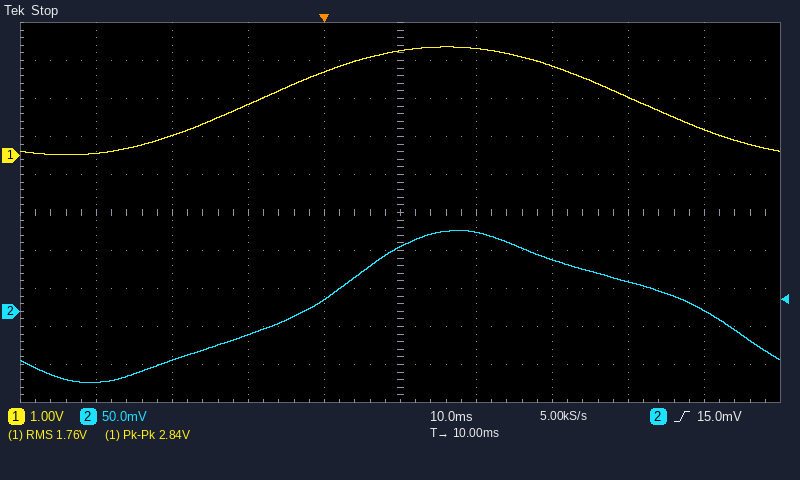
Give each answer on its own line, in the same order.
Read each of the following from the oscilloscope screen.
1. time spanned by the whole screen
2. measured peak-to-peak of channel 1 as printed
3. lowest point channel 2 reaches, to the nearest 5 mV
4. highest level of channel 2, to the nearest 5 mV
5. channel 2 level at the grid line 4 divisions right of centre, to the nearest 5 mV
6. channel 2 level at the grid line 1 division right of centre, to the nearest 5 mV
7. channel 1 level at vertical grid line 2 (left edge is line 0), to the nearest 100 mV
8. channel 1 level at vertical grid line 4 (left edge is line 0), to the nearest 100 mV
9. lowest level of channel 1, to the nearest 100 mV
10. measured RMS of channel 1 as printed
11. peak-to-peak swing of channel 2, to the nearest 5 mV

100 ms
2.84 V
-95 mV
105 mV
0 mV
105 mV
500 mV
2.2 V
0.0 V
1.76 V
200 mV
